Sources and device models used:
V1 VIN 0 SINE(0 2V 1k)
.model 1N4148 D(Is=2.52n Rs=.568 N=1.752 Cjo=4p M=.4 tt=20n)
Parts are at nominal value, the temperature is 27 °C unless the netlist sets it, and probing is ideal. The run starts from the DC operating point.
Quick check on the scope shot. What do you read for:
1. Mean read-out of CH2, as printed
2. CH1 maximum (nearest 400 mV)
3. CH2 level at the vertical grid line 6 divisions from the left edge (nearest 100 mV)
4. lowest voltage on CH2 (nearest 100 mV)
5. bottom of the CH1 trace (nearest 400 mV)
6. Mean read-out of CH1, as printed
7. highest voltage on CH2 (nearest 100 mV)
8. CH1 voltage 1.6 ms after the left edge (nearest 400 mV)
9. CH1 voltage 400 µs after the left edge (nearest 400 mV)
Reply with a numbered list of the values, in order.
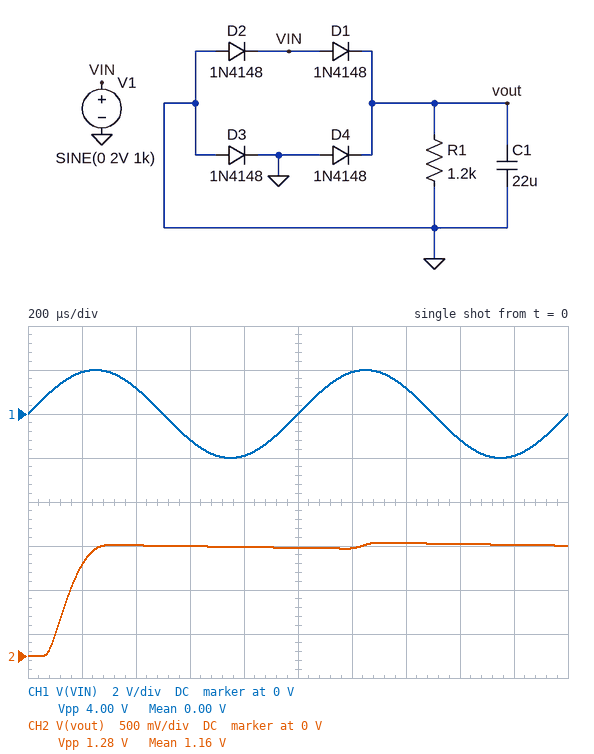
1. 1.16 V
2. 2.0 V
3. 1.2 V
4. 0 V
5. -2.0 V
6. 0.00 V
7. 1.3 V
8. -1.2 V
9. 1.2 V
